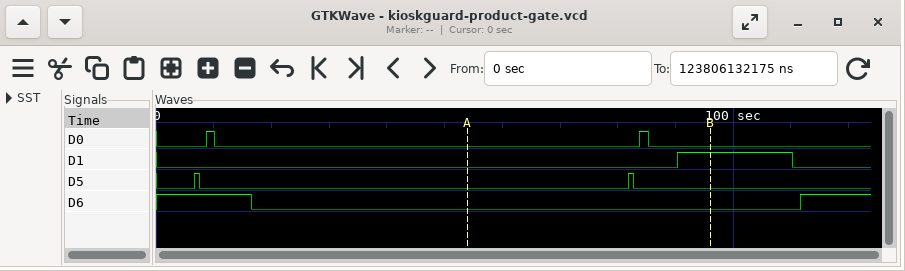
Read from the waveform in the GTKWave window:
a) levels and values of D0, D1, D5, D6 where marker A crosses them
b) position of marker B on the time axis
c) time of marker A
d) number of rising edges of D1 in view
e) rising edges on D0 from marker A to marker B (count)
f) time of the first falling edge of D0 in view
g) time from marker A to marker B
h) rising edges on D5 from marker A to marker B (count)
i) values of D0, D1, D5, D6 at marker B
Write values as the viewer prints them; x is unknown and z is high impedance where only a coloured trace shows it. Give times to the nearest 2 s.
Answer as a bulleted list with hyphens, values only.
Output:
- D0=0, D1=0, D5=0, D6=0
- 96 s
- 54 s
- 1
- 1
- 10 s
- 42 s
- 1
- D0=0, D1=1, D5=0, D6=0
